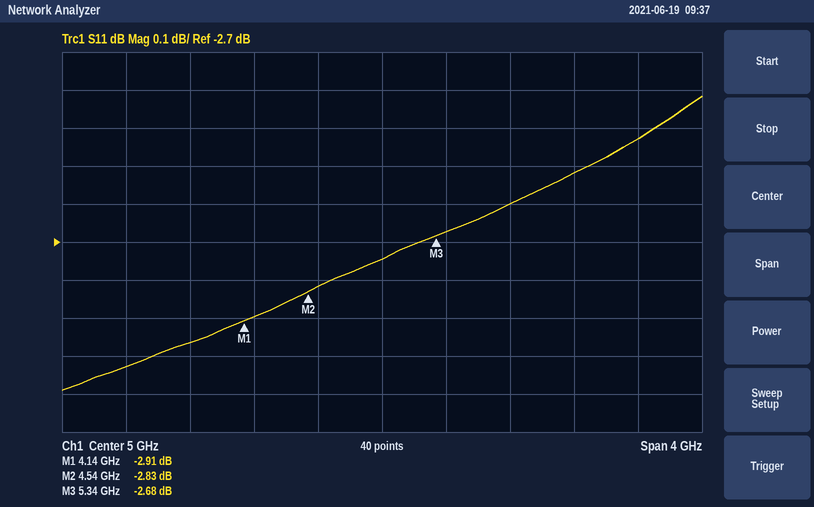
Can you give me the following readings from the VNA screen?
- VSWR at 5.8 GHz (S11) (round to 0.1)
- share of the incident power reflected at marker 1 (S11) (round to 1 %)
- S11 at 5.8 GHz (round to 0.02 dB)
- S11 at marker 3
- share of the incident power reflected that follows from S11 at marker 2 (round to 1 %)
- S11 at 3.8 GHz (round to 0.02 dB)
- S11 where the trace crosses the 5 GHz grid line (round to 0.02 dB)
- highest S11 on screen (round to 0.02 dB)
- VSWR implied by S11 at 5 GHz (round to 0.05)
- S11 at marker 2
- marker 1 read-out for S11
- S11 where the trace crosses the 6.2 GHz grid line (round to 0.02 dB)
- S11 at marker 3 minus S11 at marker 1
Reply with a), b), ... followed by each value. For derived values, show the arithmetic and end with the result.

a) |Γ| = 10^(-2.6/20) = 0.7413; VSWR = (1 + 0.7413)/(1 − 0.7413) ≈ 6.7
b) 10^(-2.91/10) ≈ 51 %
c) -2.60 dB
d) -2.68 dB
e) 10^(-2.83/10) ≈ 52 %
f) -2.96 dB
g) -2.74 dB
h) -2.32 dB
i) |Γ| = 10^(-2.74/20) = 0.7295; VSWR = (1 + 0.7295)/(1 − 0.7295) ≈ 6.39, so 6.40 to the nearest 0.05
j) -2.83 dB
k) -2.91 dB
l) -2.52 dB
m) -2.68 − (-2.91) = 0.23 dB
